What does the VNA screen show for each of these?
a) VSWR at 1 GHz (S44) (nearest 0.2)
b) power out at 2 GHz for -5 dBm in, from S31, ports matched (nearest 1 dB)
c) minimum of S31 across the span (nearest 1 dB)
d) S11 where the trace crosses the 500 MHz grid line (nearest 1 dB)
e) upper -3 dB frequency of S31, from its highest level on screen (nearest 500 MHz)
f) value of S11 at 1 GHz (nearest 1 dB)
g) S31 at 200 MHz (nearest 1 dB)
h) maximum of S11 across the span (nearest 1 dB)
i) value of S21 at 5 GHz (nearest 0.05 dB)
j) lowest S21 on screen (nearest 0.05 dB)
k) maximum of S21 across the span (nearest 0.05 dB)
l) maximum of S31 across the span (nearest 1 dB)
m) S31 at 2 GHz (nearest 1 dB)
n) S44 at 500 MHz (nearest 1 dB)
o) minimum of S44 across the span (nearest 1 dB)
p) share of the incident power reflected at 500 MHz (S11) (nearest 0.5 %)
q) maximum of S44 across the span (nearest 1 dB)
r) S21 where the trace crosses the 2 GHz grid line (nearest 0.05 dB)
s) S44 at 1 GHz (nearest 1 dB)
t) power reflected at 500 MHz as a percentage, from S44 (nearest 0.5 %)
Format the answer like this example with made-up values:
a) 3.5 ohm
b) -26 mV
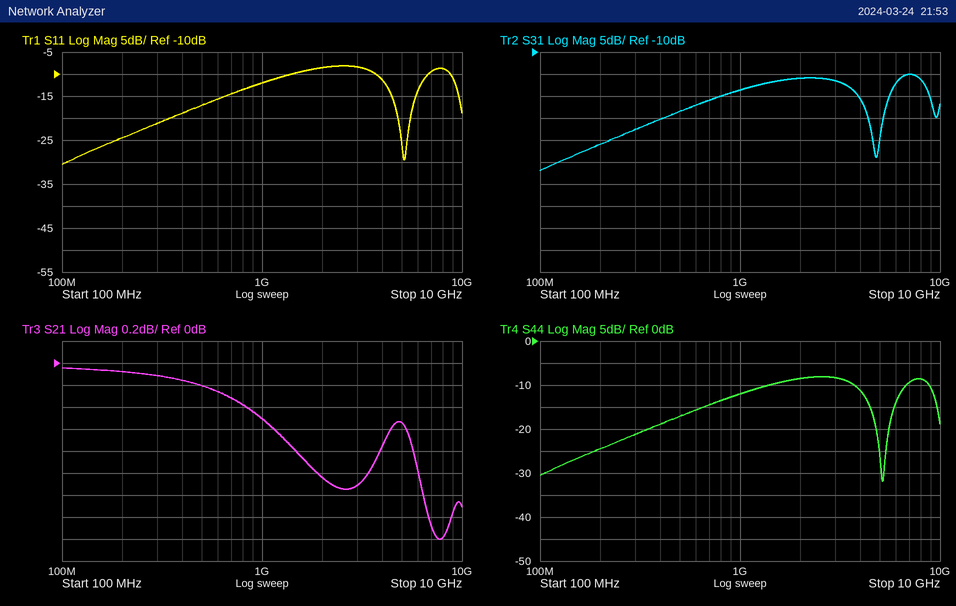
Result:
a) 1.6
b) -21 dBm
c) -37 dB
d) -17 dB
e) 8.5 GHz
f) -12 dB
g) -31 dB
h) -8 dB
i) -0.55 dB
j) -1.60 dB
k) -0.05 dB
l) -15 dB
m) -16 dB
n) -17 dB
o) -32 dB
p) 2.0 %
q) -8 dB
r) -1.05 dB
s) -12 dB
t) 2.0 %
